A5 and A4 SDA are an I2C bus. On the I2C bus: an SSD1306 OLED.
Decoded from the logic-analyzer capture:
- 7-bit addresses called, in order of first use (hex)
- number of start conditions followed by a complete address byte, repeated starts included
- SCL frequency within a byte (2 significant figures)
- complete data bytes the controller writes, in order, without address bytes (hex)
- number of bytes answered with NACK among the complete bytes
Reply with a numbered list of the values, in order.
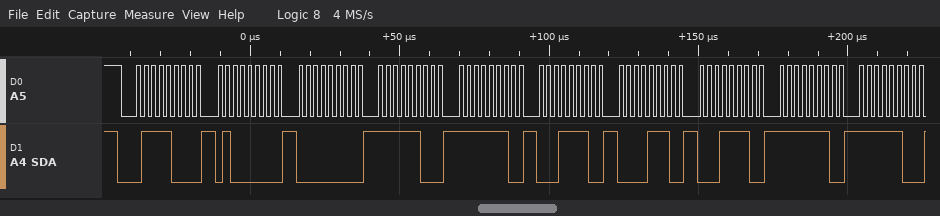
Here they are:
1. 0x3C
2. 1
3. 400 kHz
4. 40 00 FC FE 1E 0E 1E FE FC
5. 0
